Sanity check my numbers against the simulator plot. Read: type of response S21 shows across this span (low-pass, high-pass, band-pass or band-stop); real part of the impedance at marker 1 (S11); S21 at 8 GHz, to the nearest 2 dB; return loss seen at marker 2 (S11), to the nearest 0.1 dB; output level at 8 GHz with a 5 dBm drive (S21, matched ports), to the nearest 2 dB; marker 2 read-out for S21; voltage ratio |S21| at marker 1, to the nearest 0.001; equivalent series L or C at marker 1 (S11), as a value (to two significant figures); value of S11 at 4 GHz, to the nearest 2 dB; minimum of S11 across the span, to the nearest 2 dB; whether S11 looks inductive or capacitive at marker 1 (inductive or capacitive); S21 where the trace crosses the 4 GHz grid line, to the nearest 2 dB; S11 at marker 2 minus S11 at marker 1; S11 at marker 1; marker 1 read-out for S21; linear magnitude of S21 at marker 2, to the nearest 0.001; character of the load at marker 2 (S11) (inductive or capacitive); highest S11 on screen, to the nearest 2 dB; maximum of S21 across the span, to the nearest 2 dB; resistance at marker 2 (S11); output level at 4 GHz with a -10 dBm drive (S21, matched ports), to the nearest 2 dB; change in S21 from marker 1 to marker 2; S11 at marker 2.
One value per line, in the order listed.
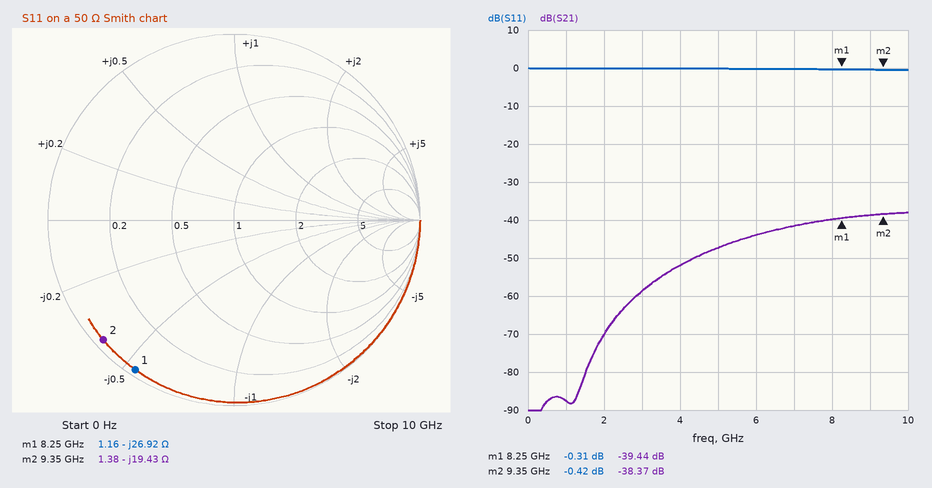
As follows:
high-pass
1.16 Ω
-40 dB
0.4 dB
-34 dBm
-38.37 dB
0.011
720 fF
0 dB
0 dB
capacitive
-52 dB
-0.11 dB
-0.31 dB
-39.44 dB
0.012
capacitive
0 dB
-38 dB
1.38 Ω
-62 dBm
1.07 dB
-0.42 dB
